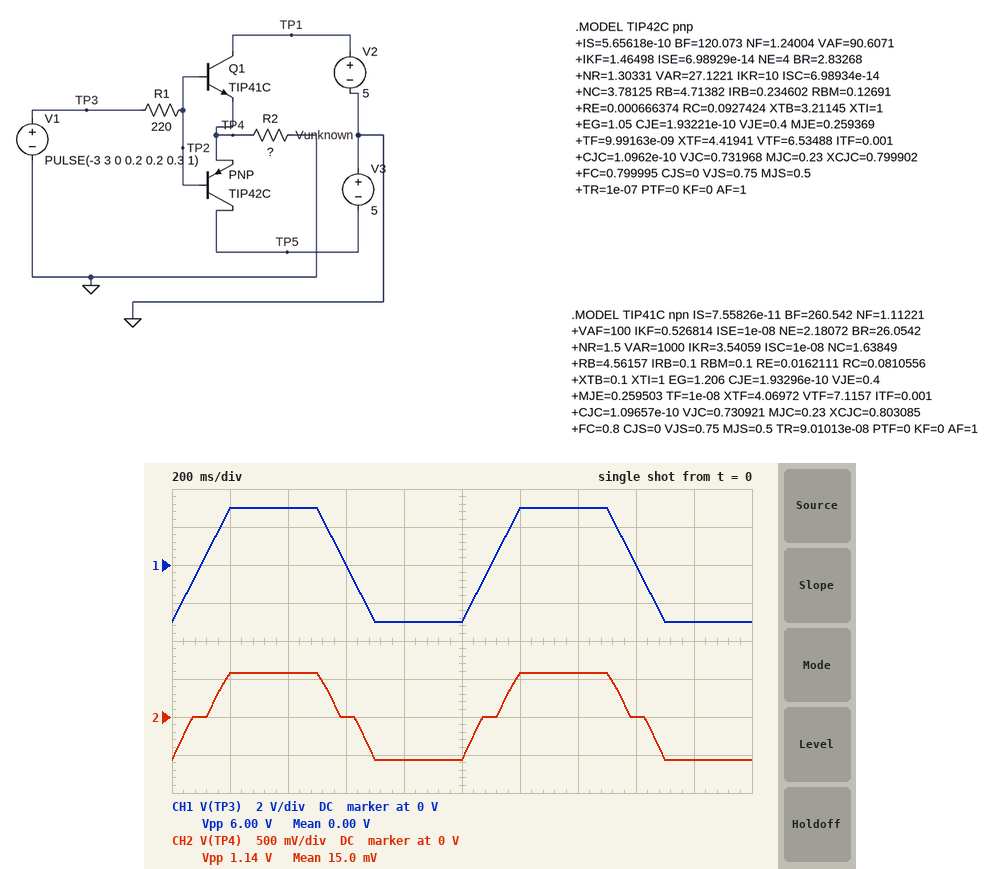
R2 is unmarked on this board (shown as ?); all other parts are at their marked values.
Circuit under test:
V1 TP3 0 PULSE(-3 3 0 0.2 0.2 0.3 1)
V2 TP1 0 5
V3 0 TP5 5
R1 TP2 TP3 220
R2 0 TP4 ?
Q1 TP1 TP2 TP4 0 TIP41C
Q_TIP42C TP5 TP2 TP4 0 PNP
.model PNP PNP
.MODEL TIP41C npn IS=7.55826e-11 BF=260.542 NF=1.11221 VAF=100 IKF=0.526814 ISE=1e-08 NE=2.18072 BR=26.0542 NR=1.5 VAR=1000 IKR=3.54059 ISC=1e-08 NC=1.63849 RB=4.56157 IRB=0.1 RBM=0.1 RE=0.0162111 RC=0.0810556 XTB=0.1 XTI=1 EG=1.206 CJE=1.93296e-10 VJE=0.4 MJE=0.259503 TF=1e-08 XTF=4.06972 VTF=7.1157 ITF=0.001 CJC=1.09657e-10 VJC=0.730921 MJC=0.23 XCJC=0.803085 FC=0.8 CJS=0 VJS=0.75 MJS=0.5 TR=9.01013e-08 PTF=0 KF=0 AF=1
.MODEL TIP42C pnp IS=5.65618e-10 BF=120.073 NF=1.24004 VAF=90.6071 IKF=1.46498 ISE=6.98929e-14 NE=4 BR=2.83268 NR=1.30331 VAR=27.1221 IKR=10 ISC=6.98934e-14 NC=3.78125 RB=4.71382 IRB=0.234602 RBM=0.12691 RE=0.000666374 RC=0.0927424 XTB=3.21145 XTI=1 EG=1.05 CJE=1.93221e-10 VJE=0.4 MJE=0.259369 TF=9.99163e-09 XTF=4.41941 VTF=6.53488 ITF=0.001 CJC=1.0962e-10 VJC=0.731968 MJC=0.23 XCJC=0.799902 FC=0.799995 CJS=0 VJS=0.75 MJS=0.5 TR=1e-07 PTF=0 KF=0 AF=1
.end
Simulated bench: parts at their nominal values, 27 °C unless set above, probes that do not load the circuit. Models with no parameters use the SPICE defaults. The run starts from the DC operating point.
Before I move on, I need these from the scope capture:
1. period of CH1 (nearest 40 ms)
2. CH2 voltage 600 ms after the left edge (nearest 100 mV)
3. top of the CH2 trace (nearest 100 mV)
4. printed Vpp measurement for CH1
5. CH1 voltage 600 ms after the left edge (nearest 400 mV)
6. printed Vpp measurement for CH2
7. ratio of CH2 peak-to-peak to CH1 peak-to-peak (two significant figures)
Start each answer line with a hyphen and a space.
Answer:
- 1.00 s
- 0 V
- 600 mV
- 6.00 V
- 0 V
- 1.14 V
- 0.19
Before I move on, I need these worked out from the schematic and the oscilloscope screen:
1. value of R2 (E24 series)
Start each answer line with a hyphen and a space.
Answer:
- 0.82 Ω
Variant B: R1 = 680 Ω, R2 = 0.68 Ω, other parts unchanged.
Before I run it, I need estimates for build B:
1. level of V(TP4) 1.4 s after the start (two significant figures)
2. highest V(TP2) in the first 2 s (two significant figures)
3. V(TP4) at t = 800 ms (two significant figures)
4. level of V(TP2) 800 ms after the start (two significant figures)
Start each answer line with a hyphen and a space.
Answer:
- 230 mV
- 900 mV
- -190 mV
- -1.1 V
